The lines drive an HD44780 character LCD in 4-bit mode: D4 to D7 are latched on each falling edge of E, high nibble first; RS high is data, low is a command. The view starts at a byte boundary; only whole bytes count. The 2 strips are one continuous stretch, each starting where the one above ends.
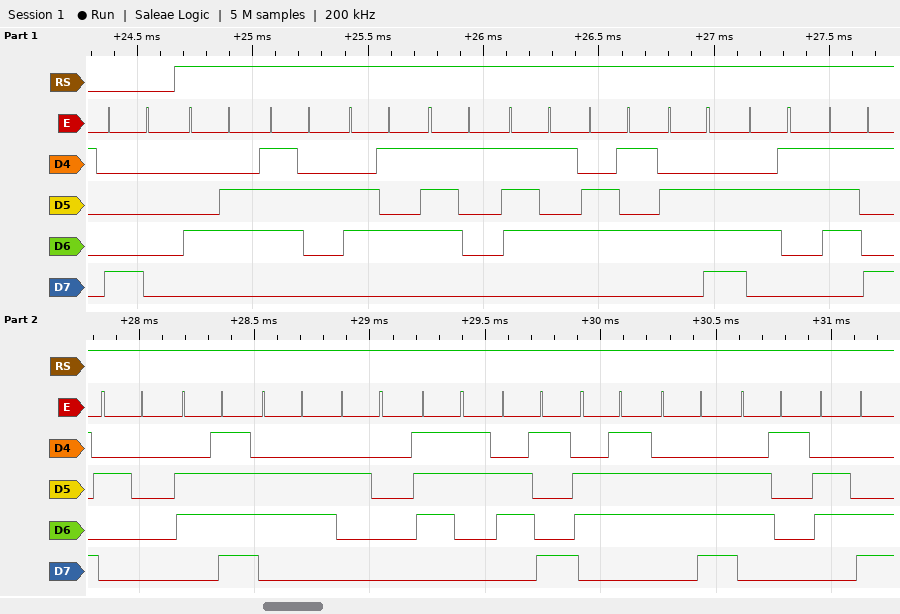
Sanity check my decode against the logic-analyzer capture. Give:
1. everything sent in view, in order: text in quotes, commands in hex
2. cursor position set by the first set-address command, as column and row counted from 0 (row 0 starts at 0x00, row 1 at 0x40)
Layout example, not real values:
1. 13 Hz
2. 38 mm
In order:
1. 0x80 "Frequency of signal"
2. column 0, row 0
